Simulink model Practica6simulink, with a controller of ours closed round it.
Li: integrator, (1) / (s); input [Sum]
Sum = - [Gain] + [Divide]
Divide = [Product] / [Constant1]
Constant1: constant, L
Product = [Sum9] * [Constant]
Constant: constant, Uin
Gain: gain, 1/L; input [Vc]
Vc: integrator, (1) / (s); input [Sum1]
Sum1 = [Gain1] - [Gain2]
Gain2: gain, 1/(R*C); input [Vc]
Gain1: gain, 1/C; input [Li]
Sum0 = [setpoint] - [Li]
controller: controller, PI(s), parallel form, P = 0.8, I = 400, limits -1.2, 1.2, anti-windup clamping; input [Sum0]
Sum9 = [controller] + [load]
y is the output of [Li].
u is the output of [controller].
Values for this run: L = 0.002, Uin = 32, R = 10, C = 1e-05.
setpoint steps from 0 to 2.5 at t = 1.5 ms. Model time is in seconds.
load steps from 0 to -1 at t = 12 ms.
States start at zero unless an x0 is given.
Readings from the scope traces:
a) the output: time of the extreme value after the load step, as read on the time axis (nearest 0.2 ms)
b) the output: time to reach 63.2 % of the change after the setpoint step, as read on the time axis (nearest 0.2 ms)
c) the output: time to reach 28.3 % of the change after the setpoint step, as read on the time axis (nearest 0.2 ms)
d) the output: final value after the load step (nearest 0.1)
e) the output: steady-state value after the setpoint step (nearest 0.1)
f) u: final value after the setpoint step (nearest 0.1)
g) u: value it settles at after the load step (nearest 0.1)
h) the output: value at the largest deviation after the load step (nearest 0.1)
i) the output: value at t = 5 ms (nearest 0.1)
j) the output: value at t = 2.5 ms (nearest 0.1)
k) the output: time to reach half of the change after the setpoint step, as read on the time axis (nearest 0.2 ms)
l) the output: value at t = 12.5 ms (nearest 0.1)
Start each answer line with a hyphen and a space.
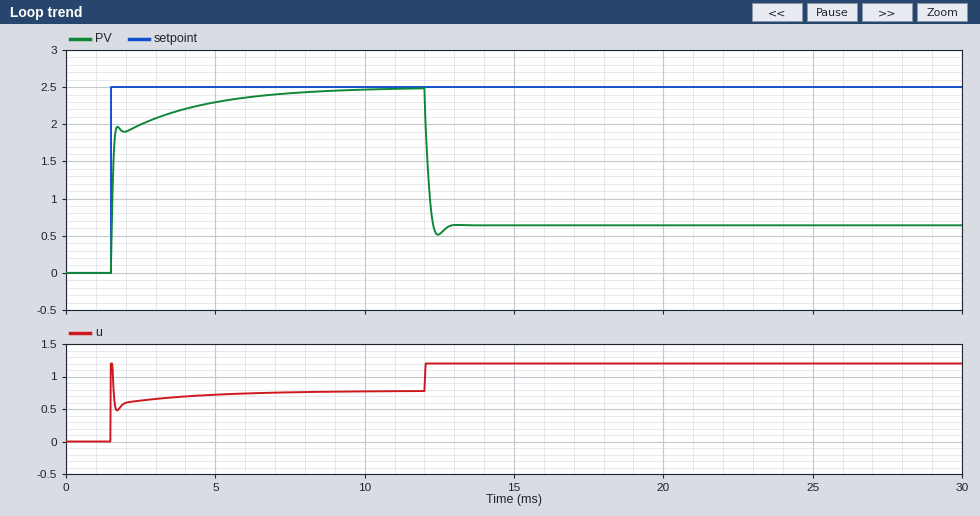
- 12.4 ms
- 1.6 ms
- 1.6 ms
- 0.6
- 2.5
- 0.8
- 1.2
- 0.5
- 2.3
- 2.0
- 1.6 ms
- 0.5
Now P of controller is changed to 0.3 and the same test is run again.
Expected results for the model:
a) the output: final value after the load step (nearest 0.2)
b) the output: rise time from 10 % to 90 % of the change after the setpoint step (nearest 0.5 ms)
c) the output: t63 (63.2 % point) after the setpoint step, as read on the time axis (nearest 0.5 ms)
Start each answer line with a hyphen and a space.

- 0.6
- 2.5 ms
- 2.0 ms
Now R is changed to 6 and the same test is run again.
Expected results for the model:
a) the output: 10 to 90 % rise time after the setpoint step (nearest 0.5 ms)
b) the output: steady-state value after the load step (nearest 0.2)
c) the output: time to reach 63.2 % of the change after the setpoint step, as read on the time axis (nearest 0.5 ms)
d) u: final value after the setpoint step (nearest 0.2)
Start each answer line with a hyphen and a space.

- 1.5 ms
- 1.0
- 1.5 ms
- 0.4
